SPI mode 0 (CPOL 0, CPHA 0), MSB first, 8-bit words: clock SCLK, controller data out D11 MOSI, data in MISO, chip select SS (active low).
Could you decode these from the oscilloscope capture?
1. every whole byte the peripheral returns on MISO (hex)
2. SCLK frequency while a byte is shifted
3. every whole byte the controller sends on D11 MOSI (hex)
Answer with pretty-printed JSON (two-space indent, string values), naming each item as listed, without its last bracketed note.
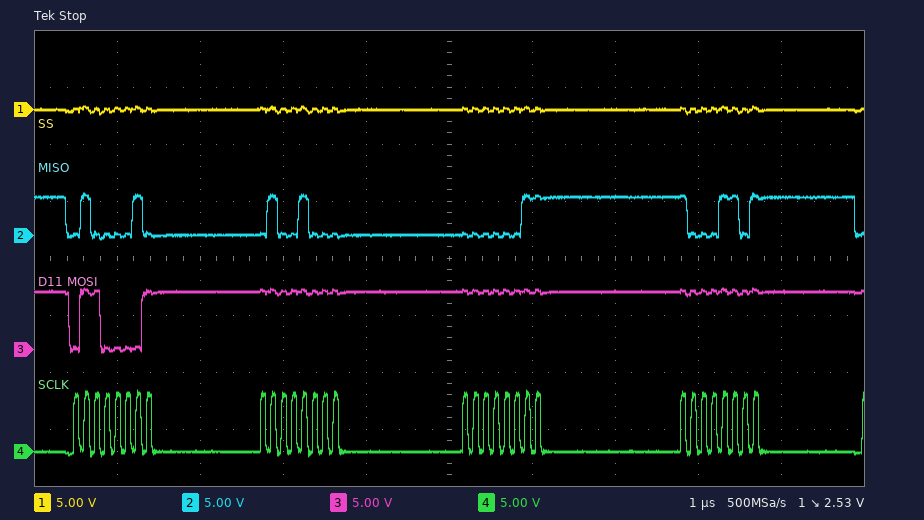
{
  "every whole byte the peripheral returns on MISO": "42 48 03 8D",
  "SCLK frequency while a byte is shifted": "8 MHz",
  "every whole byte the controller sends on D11 MOSI": "61 FF FF FF"
}
